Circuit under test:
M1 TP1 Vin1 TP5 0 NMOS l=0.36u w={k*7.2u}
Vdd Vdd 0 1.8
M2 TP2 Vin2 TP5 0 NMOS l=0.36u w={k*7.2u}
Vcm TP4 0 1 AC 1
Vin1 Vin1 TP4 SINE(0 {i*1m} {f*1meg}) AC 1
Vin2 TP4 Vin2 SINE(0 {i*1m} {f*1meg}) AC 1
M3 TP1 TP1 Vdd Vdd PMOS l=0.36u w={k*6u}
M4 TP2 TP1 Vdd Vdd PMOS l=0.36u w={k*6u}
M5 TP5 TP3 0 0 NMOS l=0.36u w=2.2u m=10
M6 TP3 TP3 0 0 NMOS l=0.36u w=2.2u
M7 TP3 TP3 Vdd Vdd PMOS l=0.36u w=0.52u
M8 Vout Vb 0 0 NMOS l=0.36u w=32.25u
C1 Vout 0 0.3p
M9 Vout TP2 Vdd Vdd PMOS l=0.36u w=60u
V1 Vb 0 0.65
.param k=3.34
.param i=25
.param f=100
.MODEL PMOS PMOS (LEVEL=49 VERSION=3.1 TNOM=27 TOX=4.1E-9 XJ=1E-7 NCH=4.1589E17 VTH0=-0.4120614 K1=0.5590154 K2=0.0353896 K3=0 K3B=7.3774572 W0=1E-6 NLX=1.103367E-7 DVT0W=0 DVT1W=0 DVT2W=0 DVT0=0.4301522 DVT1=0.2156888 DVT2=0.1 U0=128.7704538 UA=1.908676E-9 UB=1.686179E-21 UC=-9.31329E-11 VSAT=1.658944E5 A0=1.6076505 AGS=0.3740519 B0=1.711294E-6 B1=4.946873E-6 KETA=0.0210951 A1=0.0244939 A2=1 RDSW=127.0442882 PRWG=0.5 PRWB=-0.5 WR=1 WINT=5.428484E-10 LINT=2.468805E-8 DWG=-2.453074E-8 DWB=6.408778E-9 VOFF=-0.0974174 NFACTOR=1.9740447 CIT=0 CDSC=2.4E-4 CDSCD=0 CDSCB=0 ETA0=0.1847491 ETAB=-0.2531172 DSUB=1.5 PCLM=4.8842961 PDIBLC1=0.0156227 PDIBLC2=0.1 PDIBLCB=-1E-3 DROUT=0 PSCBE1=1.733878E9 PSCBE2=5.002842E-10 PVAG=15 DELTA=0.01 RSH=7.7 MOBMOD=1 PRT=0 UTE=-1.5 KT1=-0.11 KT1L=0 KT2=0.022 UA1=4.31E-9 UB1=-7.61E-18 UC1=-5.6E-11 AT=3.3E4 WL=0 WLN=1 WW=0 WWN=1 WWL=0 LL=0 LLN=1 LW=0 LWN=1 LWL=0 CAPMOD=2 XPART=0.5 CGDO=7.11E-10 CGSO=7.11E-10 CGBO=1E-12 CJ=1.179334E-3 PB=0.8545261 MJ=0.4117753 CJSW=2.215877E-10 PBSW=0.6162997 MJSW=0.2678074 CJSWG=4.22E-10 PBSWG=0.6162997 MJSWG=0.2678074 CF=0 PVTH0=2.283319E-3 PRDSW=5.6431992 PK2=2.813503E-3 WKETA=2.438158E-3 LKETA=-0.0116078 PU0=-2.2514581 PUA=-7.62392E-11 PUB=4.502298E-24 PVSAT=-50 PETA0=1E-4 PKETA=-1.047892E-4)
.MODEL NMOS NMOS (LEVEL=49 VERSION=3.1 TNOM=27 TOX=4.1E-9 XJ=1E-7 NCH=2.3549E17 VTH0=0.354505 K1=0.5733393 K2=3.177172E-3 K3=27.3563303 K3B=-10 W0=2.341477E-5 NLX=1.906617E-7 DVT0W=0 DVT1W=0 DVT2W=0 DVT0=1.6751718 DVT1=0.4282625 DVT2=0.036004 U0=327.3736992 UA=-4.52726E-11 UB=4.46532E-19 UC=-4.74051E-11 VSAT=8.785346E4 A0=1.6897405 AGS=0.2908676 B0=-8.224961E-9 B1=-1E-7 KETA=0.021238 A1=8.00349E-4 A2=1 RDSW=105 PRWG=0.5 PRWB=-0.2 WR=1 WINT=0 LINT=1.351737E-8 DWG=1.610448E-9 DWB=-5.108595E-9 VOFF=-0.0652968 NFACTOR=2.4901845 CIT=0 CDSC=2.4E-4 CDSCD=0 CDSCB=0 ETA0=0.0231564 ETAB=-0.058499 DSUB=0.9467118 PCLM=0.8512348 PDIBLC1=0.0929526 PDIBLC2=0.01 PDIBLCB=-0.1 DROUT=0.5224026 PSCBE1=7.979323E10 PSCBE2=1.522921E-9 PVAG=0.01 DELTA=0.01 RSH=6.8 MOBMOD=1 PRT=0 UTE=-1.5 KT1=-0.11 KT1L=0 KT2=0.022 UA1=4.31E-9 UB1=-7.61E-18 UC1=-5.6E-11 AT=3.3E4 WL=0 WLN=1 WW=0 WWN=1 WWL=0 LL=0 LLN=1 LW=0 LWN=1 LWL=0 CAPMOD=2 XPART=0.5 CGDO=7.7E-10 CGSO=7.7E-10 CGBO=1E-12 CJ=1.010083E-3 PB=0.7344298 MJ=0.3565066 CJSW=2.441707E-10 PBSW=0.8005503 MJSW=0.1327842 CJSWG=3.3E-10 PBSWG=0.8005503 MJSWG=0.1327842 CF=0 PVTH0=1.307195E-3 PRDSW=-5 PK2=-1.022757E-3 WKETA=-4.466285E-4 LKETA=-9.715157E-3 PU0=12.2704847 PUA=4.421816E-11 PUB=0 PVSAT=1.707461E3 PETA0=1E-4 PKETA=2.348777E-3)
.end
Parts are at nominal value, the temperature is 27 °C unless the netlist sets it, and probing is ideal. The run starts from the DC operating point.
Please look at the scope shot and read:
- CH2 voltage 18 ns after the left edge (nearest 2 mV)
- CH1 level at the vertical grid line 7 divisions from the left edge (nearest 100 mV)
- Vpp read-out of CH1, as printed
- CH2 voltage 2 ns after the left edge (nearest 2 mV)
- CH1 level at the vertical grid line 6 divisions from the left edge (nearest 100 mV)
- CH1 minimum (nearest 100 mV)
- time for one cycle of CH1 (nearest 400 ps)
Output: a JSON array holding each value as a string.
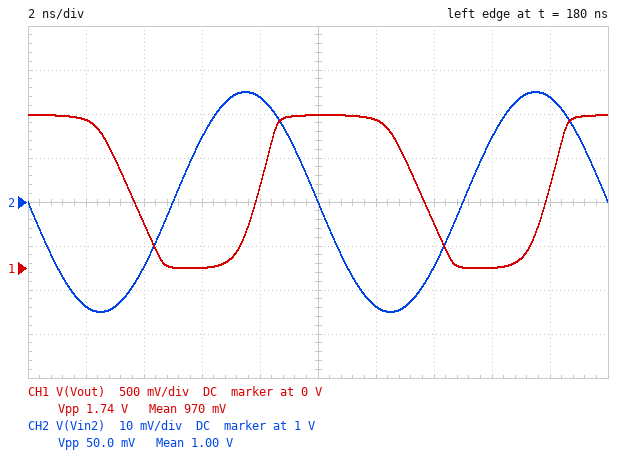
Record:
["1.024 V", "500 mV", "1.74 V", "976 mV", "1.7 V", "0 V", "10.0 ns"]
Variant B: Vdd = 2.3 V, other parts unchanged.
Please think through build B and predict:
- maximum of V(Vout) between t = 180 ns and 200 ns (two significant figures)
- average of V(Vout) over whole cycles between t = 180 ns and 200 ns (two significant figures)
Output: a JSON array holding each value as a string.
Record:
["2.3 V", "1.5 V"]
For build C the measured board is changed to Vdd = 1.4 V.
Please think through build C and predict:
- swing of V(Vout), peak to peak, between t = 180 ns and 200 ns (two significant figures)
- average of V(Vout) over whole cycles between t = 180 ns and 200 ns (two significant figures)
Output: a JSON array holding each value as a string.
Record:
["530 mV", "160 mV"]
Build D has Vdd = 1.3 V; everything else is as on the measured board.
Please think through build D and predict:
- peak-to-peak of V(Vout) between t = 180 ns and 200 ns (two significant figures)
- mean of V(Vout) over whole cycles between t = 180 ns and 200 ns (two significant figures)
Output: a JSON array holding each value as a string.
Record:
["110 mV", "36 mV"]
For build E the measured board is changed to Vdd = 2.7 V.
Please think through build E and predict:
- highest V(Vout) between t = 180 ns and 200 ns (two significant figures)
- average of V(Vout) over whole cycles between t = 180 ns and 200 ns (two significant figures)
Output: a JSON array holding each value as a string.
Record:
["2.7 V", "2.0 V"]
